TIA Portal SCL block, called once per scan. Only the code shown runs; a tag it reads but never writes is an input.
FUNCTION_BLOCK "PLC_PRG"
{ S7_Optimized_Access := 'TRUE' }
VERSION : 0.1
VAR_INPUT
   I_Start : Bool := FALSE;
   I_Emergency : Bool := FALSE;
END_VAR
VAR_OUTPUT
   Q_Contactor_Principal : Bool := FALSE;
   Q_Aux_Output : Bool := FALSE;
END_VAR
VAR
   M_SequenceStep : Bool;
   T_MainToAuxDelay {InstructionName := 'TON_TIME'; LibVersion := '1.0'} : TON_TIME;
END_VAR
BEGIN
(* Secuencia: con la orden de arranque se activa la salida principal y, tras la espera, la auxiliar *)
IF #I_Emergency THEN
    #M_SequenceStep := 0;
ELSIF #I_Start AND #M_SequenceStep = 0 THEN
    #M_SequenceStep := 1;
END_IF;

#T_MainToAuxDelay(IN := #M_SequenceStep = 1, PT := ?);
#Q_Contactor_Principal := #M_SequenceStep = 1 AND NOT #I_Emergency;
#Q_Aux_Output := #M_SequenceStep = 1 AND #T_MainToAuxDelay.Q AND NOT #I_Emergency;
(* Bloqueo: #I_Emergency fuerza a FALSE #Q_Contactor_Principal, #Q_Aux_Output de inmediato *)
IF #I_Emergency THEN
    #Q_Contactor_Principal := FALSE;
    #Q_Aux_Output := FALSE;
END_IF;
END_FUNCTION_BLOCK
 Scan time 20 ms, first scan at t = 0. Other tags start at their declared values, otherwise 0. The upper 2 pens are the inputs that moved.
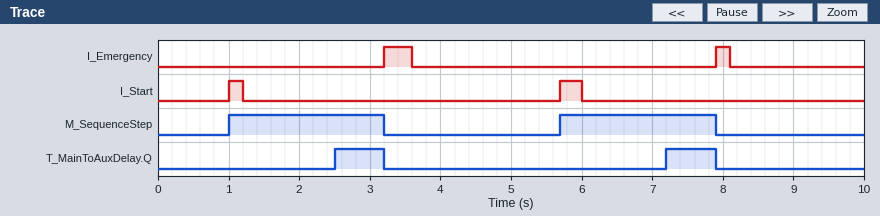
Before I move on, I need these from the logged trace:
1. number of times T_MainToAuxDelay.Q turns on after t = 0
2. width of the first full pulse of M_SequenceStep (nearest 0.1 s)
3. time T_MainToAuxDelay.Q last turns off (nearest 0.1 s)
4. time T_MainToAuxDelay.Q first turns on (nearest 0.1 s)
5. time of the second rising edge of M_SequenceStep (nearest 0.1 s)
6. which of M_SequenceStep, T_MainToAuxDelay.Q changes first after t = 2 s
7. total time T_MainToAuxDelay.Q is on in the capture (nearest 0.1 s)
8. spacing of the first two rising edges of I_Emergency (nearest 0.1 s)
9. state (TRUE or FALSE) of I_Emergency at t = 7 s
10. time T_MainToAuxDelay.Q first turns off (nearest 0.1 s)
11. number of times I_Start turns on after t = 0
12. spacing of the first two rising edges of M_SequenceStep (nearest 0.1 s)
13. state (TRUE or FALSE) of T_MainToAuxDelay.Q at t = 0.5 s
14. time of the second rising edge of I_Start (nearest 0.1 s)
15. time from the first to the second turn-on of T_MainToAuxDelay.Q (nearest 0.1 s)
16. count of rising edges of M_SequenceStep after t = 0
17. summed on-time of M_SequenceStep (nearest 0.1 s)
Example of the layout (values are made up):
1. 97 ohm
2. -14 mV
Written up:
1. 2
2. 2.2 s
3. 7.9 s
4. 2.5 s
5. 5.7 s
6. T_MainToAuxDelay.Q
7. 1.4 s
8. 4.7 s
9. FALSE
10. 3.2 s
11. 2
12. 4.7 s
13. FALSE
14. 5.7 s
15. 4.7 s
16. 2
17. 4.4 s
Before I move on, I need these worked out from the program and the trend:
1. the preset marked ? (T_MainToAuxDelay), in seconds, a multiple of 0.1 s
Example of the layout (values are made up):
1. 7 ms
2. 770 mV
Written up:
1. 1.5 s
